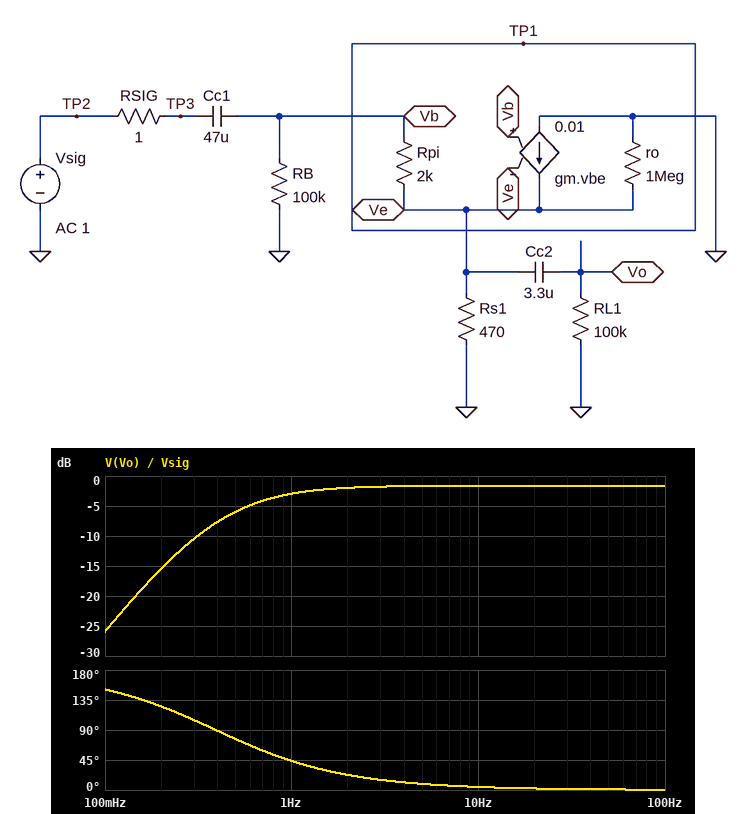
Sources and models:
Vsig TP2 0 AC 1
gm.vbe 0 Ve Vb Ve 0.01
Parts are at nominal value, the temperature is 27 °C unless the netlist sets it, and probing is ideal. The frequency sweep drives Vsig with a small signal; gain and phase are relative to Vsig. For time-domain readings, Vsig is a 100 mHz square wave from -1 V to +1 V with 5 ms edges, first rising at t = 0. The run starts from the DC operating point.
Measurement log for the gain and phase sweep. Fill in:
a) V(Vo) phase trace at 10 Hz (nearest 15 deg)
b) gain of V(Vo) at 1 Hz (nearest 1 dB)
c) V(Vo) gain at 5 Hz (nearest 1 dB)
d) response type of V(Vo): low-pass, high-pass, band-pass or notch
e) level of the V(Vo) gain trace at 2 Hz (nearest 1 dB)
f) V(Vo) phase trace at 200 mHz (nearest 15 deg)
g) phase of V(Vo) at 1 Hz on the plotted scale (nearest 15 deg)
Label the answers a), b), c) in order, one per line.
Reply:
a) 0 deg
b) -3 dB
c) -2 dB
d) high-pass
e) -2 dB
f) 120 deg
g) 45 deg
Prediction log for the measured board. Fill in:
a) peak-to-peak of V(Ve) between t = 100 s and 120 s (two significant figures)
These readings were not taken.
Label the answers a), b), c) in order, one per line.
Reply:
a) 3.3 V
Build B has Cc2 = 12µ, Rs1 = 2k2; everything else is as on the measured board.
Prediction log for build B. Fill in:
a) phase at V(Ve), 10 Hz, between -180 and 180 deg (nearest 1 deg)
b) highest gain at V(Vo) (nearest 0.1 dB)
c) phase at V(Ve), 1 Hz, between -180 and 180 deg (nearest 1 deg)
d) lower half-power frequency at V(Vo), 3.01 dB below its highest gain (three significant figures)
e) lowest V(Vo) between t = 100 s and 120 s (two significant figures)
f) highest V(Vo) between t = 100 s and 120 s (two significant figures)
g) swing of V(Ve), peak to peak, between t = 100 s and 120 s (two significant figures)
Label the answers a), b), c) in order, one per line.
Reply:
a) 1 deg
b) -0.4 dB
c) 6 deg
d) 186 mHz
e) -2.0 V
f) 2.0 V
g) 3.7 V
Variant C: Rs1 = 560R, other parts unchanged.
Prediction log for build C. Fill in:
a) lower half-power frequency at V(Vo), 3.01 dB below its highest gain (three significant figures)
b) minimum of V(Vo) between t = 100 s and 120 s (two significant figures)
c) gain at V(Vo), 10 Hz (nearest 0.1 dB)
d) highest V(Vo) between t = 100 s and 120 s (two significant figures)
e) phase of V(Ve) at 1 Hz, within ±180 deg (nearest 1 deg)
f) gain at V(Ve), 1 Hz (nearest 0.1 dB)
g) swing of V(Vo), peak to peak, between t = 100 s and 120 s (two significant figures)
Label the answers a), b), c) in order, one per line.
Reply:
a) 602 mHz
b) -1.7 V
c) -1.4 dB
d) 1.7 V
e) 16 deg
f) -1.7 dB
g) 3.4 V
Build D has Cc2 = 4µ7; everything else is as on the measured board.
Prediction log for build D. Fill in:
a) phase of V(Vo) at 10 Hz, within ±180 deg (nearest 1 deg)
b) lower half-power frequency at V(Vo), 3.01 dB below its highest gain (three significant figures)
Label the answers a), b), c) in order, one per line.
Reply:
a) 4 deg
b) 512 mHz
